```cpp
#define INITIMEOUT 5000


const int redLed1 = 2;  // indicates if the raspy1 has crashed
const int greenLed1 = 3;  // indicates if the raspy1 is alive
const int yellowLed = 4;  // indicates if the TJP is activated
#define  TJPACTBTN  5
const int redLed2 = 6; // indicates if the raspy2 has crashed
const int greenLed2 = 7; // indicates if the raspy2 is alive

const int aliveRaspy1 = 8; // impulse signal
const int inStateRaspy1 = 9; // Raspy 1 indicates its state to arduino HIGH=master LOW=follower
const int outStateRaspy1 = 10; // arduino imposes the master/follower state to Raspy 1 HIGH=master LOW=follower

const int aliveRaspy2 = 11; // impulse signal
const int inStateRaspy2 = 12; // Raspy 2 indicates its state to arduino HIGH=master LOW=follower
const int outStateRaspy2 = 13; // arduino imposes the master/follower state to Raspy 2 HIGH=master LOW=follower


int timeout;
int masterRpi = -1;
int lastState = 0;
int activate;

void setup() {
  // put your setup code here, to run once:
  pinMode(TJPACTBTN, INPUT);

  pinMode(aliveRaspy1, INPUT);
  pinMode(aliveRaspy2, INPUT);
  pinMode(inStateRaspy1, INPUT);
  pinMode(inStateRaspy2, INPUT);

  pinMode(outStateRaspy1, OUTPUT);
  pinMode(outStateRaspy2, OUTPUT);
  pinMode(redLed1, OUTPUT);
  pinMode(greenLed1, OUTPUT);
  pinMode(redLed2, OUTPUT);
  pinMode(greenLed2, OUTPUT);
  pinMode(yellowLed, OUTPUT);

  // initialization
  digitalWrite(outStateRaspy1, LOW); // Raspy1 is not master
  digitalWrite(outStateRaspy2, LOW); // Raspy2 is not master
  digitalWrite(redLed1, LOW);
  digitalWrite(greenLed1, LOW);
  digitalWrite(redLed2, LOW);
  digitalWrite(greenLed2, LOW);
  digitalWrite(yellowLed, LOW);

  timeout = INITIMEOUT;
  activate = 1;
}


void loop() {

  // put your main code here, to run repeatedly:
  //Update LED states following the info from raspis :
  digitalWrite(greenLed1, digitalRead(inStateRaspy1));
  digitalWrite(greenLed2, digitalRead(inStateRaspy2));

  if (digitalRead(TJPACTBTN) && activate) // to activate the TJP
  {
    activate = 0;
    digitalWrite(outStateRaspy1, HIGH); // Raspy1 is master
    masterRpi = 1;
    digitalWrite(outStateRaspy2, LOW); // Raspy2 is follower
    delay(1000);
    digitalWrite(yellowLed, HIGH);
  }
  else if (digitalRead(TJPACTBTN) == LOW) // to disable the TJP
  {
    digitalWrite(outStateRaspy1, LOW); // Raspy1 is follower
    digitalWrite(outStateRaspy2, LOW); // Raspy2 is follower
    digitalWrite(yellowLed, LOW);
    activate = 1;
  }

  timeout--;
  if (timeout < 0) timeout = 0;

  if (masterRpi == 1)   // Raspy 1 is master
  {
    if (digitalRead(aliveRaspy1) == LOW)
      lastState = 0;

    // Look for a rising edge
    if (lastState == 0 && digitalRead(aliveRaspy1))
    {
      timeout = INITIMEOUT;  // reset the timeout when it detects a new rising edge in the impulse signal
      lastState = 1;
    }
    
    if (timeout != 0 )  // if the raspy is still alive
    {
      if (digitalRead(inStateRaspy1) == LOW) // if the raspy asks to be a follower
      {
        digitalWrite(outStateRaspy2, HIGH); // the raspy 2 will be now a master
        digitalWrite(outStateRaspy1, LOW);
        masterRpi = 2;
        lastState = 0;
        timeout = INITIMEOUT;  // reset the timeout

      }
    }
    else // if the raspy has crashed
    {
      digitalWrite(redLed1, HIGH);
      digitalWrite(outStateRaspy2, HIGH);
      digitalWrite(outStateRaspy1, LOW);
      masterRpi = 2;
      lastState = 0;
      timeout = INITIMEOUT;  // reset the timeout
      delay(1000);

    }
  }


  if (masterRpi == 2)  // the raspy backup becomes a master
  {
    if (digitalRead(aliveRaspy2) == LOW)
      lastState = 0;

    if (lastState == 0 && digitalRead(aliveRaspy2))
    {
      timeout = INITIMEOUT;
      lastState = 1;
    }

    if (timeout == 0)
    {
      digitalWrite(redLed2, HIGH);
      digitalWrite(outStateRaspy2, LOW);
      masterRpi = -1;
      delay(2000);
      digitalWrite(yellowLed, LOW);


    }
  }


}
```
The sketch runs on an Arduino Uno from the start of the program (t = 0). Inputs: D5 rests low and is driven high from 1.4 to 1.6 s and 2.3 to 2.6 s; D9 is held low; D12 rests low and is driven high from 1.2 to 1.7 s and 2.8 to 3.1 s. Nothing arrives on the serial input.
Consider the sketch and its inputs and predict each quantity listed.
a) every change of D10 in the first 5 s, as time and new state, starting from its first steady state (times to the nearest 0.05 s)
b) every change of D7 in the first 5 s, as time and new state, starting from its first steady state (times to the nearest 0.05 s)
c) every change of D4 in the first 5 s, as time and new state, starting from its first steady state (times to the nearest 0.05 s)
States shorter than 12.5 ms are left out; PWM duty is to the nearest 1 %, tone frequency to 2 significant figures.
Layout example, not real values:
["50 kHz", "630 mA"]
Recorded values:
["0 s low; 1.4 s high; 2.4 s low", "0 s low; 1.2 s high; 3.4 s low", "0 s low; 2.4 s high; 3.4 s low"]
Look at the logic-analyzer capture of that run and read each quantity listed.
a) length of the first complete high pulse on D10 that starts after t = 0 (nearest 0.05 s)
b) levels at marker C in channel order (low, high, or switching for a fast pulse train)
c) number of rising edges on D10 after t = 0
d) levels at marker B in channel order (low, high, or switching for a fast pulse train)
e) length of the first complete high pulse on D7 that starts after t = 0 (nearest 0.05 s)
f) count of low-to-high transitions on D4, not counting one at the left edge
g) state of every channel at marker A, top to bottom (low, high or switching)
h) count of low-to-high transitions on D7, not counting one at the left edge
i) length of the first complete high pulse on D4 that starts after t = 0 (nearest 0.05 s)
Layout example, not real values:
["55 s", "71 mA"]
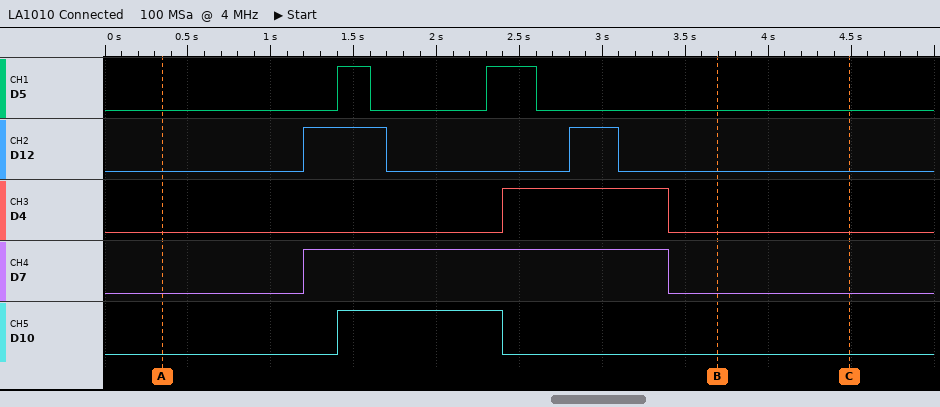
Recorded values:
["1.00 s", "D5 low, D12 low, D4 low, D7 low, D10 low", "1", "D5 low, D12 low, D4 low, D7 low, D10 low", "2.20 s", "1", "D5 low, D12 low, D4 low, D7 low, D10 low", "1", "1.00 s"]
